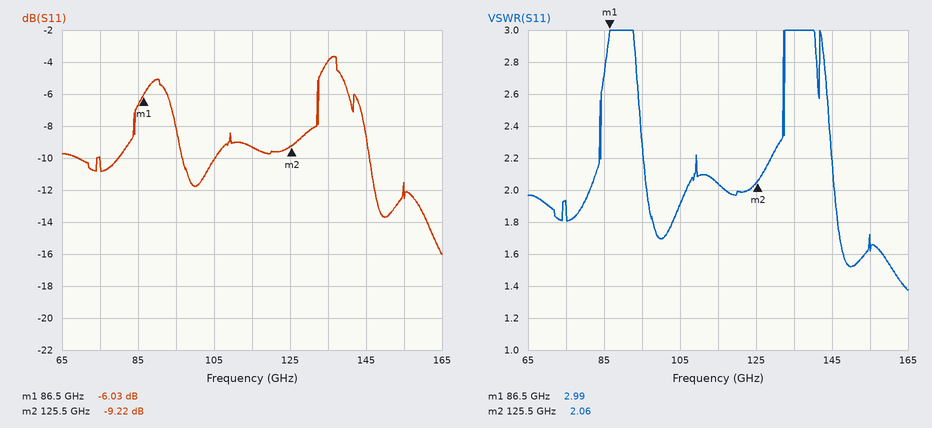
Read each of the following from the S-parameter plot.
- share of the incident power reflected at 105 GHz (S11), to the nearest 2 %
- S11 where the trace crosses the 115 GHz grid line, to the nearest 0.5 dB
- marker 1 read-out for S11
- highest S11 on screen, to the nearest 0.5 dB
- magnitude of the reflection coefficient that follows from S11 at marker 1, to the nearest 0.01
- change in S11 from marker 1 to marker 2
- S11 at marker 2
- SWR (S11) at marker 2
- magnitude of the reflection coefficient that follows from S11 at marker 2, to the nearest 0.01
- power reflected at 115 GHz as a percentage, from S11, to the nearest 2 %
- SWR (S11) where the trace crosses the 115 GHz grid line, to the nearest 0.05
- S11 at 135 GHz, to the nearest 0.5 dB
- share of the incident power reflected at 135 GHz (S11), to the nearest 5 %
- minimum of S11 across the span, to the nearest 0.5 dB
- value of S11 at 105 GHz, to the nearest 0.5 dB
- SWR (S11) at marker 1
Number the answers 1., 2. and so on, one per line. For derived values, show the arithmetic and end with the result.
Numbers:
1. 10^(-10/10) ≈ 10 %
2. -9.5 dB
3. -6.03 dB
4. -3.5 dB
5. 10^(-6.03/20) ≈ 0.50
6. -9.22 − (-6.03) = -3.19 dB
7. -9.22 dB
8. 2.06
9. 10^(-9.22/20) ≈ 0.35
10. 10^(-9.5/10) ≈ 11.2 %, so 12 % to the nearest 2 %
11. 2.05
12. -4.0 dB
13. 10^(-4/10) ≈ 40 %
14. -16.0 dB
15. -10.0 dB
16. 2.99
